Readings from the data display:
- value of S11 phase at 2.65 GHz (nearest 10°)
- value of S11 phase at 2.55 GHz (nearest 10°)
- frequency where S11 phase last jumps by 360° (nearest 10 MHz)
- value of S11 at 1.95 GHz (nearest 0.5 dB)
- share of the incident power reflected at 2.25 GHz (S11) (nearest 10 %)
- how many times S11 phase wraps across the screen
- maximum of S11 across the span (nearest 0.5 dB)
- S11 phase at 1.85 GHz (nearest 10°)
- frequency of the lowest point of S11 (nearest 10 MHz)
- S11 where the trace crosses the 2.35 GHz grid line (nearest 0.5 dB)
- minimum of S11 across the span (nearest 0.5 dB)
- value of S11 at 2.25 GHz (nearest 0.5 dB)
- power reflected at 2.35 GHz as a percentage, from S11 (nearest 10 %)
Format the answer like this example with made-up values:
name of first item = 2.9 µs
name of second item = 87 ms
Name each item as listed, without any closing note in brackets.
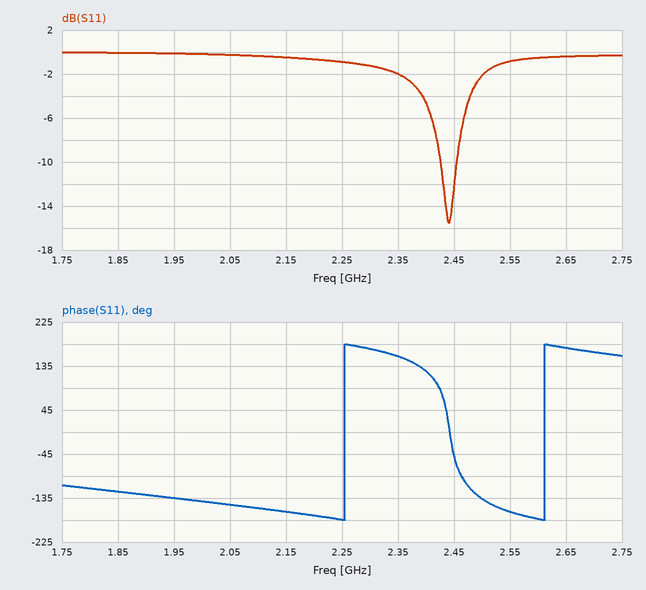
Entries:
value of S11 phase at 2.65 GHz = 170°
value of S11 phase at 2.55 GHz = -160°
frequency where S11 phase last jumps by 360° = 2.61 GHz
value of S11 at 1.95 GHz = 0.0 dB
share of the incident power reflected at 2.25 GHz (S11) = 80 %
how many times S11 phase wraps across the screen = 2
maximum of S11 across the span = 0.0 dB
S11 phase at 1.85 GHz = -120°
frequency of the lowest point of S11 = 2.44 GHz
S11 where the trace crosses the 2.35 GHz grid line = -2.0 dB
minimum of S11 across the span = -15.5 dB
value of S11 at 2.25 GHz = -1.0 dB
power reflected at 2.35 GHz as a percentage, from S11 = 60 %
